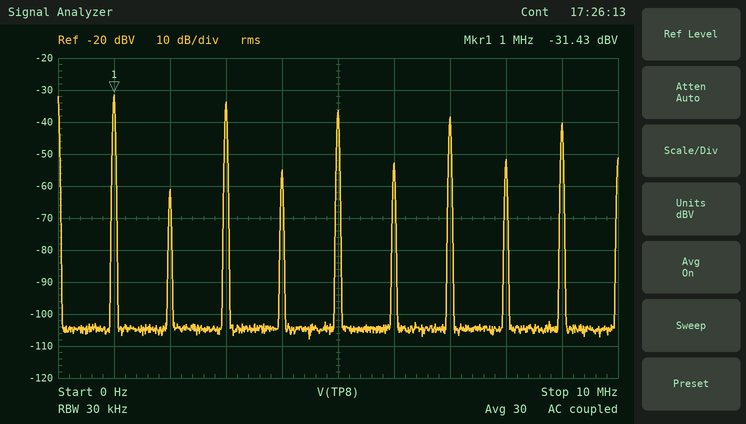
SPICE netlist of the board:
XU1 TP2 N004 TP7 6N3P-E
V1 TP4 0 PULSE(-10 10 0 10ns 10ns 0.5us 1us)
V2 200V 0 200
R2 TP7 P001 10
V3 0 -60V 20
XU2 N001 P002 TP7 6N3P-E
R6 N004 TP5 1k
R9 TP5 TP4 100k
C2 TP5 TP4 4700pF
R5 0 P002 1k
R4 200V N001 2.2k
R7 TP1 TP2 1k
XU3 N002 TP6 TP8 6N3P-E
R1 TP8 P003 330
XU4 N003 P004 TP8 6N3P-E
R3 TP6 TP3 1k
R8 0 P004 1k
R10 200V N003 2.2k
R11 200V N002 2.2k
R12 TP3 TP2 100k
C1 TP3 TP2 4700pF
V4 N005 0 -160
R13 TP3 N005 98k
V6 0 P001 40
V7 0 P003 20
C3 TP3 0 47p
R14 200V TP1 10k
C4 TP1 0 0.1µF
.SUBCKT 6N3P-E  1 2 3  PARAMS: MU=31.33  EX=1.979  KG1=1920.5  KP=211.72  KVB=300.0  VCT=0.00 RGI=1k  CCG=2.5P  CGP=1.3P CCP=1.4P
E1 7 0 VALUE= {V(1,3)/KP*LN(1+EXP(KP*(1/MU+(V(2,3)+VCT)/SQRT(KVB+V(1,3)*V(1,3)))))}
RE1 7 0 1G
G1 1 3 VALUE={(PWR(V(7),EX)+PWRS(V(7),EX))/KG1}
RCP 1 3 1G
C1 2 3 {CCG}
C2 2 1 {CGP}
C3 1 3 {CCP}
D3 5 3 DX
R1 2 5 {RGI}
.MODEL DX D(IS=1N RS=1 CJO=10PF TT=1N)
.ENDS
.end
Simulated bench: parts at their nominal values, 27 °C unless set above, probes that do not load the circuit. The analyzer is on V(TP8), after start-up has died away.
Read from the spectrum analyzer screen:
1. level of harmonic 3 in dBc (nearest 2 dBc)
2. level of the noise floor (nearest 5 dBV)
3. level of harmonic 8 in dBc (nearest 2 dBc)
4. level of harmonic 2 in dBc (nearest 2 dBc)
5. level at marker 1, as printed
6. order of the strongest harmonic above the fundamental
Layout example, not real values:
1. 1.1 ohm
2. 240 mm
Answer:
1. -2 dBc
2. -105 dBV
3. -20 dBc
4. -30 dBc
5. -31.43 dBV
6. 3
